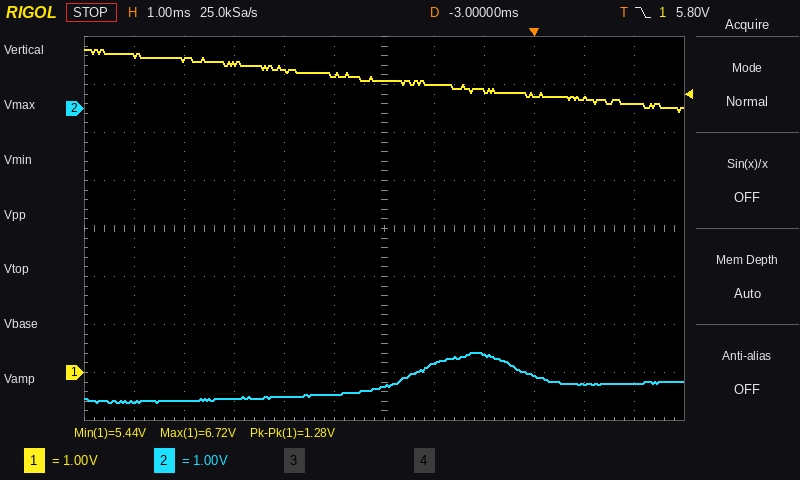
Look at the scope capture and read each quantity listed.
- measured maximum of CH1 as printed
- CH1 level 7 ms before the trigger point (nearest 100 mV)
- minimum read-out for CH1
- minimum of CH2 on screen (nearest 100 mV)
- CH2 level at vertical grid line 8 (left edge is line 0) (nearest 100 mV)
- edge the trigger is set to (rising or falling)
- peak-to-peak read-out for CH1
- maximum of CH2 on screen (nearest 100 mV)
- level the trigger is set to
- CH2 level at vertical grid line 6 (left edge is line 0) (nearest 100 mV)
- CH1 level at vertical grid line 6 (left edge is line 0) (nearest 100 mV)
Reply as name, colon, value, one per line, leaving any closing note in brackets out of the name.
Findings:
measured maximum of CH1 as printed: 6.72 V
CH1 level 7 ms before the trigger point: 6.5 V
minimum read-out for CH1: 5.44 V
minimum of CH2 on screen: -6.1 V
CH2 level at vertical grid line 8 (left edge is line 0): -5.1 V
edge the trigger is set to: falling
peak-to-peak read-out for CH1: 1.28 V
maximum of CH2 on screen: -5.1 V
level the trigger is set to: 5.80 V
CH2 level at vertical grid line 6 (left edge is line 0): -5.8 V
CH1 level at vertical grid line 6 (left edge is line 0): 6.1 V
